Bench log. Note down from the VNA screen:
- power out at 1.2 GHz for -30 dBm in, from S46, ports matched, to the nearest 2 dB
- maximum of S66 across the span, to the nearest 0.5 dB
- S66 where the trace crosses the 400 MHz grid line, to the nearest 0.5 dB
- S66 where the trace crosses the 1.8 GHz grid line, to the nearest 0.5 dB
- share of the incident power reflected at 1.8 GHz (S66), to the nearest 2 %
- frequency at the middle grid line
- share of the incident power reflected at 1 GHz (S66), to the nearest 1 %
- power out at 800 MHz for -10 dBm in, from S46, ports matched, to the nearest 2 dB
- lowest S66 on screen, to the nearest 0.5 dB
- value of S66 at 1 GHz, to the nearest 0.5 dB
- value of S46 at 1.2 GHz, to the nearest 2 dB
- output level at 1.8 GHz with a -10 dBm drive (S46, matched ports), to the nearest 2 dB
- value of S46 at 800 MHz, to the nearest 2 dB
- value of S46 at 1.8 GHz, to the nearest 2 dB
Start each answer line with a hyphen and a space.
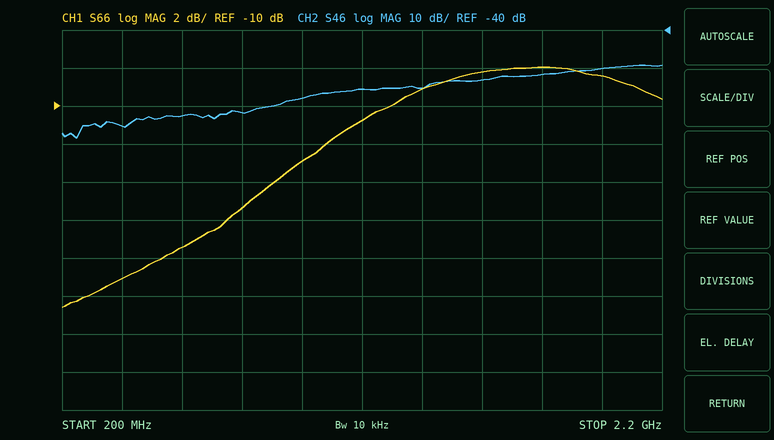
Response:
- -86 dBm
- -8.0 dB
- -19.0 dB
- -8.0 dB
- 16 %
- 1.2 GHz
- 5 %
- -72 dBm
- -20.5 dB
- -13.0 dB
- -56 dB
- -62 dBm
- -62 dB
- -52 dB
